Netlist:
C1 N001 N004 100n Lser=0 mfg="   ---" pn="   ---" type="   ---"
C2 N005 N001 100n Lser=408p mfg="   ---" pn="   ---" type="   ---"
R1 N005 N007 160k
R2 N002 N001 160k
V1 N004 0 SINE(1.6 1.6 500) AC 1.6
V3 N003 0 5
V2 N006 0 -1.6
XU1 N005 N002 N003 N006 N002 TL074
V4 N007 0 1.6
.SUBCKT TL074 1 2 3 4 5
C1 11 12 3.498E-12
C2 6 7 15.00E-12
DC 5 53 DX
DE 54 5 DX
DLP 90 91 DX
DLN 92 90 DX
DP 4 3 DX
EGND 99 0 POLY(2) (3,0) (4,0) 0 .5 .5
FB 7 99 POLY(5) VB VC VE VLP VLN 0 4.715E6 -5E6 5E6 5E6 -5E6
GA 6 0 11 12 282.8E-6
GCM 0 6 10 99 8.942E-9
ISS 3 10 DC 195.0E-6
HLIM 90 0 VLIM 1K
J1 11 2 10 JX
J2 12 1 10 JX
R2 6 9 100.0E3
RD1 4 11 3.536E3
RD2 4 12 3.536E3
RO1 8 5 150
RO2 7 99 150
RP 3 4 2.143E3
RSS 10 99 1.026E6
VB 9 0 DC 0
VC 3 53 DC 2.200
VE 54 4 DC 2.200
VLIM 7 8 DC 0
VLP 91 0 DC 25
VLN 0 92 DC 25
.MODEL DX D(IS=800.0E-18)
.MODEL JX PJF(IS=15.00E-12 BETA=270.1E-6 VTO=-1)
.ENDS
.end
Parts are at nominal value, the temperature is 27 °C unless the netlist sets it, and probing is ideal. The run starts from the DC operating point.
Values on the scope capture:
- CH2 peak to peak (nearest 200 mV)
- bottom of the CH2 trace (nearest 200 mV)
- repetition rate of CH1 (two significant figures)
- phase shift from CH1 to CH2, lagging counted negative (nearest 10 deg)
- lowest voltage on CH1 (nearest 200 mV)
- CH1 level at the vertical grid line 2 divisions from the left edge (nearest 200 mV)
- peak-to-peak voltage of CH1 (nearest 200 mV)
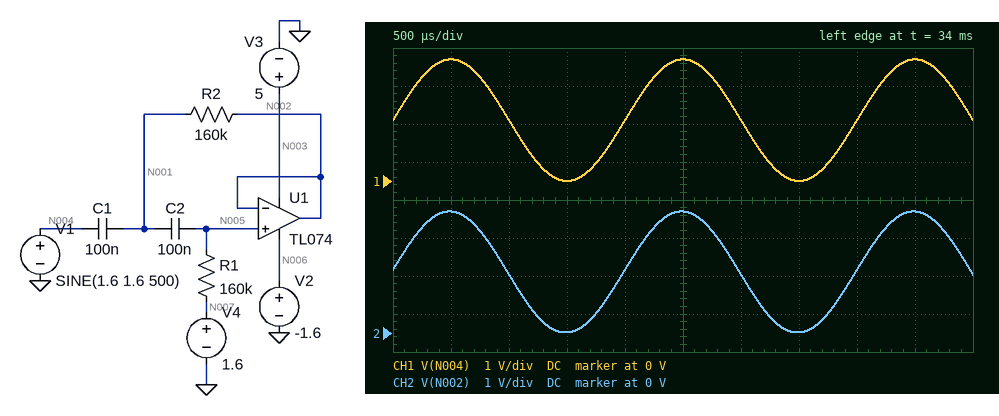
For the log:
3.2 V
0 V
500 Hz
0 deg
0 V
1.6 V
3.2 V
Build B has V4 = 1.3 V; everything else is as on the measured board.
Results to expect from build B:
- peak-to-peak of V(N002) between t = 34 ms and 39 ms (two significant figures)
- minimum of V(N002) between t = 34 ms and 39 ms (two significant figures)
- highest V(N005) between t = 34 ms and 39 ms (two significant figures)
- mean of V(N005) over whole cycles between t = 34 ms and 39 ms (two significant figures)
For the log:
3.0 V
-51 mV
2.9 V
1.3 V
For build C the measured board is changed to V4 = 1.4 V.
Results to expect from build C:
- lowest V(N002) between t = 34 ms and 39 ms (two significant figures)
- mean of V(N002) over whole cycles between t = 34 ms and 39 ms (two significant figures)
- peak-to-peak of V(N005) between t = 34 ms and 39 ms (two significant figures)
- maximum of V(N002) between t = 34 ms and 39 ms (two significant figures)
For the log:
-41 mV
1.4 V
3.2 V
3.0 V
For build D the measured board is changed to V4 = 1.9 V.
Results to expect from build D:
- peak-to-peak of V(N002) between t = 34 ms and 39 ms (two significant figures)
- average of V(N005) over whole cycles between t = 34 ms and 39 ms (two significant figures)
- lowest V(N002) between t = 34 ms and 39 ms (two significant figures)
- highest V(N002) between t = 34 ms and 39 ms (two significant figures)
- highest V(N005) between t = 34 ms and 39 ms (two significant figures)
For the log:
3.1 V
1.9 V
300 mV
3.4 V
3.5 V
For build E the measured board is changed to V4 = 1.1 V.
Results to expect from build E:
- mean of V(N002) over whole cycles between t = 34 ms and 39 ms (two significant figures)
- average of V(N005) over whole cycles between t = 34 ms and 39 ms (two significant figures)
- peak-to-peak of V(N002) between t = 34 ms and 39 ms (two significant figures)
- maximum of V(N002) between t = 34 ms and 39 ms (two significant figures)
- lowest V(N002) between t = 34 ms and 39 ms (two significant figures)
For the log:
1.2 V
1.1 V
2.8 V
2.7 V
-59 mV
